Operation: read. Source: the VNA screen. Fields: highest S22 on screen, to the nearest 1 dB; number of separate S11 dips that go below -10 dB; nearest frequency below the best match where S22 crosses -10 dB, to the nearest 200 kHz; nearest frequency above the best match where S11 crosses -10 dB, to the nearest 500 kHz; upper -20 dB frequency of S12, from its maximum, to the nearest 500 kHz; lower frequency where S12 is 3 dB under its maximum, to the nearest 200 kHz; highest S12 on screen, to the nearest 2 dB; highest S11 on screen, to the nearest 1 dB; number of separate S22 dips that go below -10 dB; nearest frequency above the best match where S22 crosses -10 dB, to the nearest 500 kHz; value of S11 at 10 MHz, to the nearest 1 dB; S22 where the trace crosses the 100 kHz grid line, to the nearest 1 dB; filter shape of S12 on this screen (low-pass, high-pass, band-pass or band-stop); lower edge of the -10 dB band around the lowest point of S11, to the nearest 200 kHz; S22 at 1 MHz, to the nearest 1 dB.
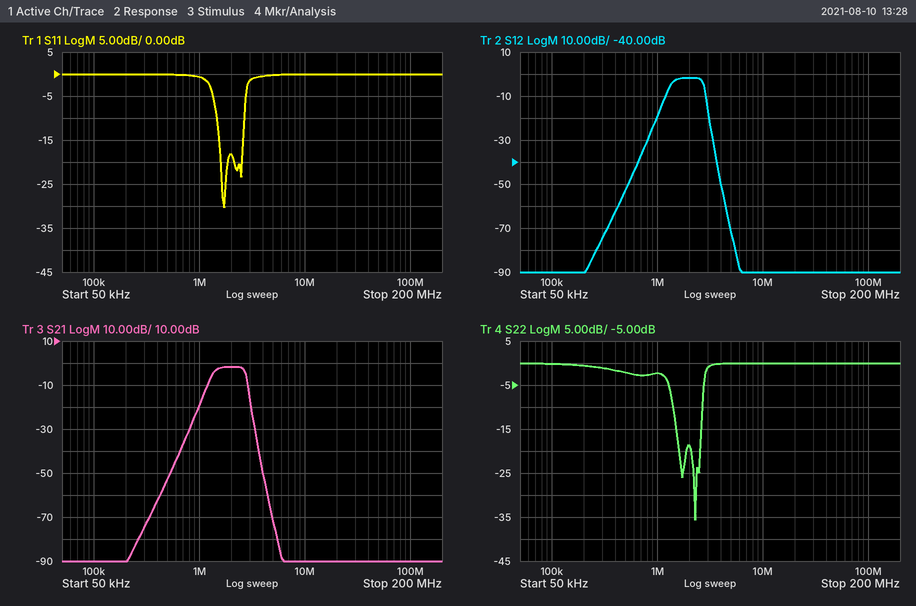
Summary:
0 dB
2
1.4 MHz
2.5 MHz
3.0 MHz
1.4 MHz
-2 dB
0 dB
2
2.5 MHz
0 dB
0 dB
band-pass
1.4 MHz
-2 dB
